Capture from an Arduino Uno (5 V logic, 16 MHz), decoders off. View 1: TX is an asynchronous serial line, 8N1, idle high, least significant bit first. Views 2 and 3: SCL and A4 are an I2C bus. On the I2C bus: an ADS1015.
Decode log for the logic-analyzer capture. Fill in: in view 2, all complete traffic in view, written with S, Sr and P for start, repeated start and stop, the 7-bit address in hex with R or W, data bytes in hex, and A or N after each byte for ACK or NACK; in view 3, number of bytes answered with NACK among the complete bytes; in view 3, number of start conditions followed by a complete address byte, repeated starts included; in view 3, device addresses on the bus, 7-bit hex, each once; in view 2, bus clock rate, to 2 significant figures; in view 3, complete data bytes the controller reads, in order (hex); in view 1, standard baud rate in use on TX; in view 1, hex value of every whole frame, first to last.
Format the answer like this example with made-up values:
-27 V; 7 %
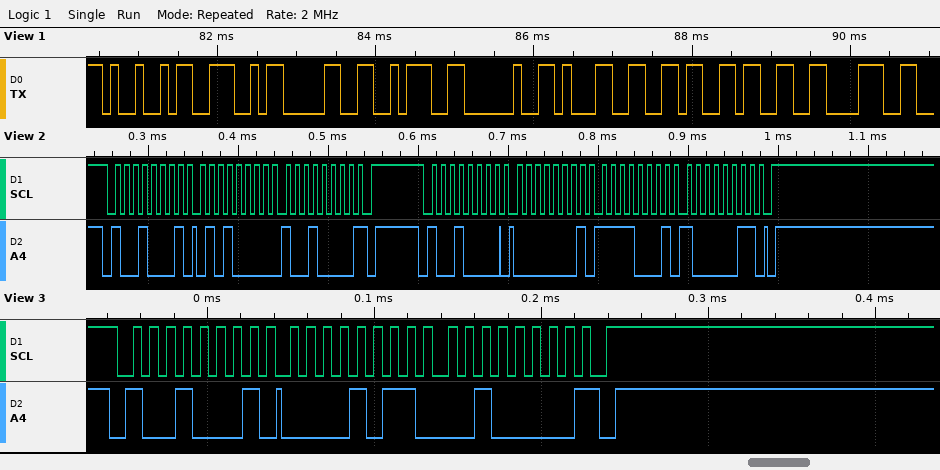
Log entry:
S 48R A 50 A 90 N P S 48W A 01 A F1 A 83 A P; 1; 1; 0x48; 100 kHz; 0B 20; 9600 baud; 49 4E 30 3A 20 31 36 33 38
